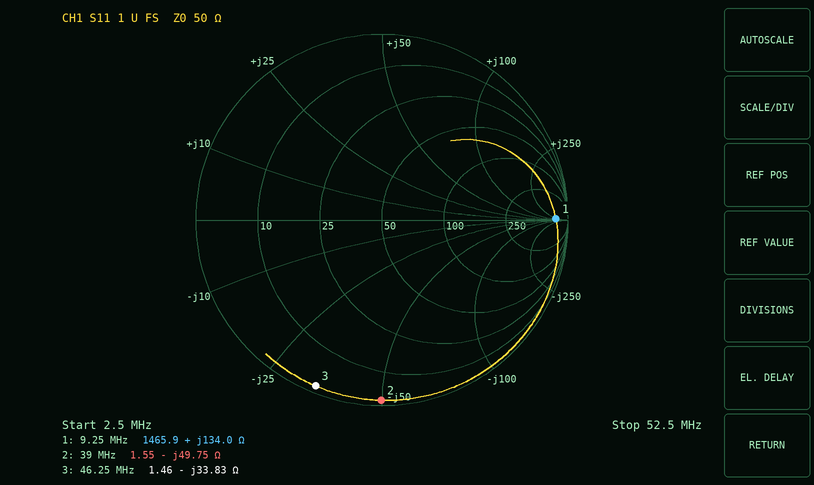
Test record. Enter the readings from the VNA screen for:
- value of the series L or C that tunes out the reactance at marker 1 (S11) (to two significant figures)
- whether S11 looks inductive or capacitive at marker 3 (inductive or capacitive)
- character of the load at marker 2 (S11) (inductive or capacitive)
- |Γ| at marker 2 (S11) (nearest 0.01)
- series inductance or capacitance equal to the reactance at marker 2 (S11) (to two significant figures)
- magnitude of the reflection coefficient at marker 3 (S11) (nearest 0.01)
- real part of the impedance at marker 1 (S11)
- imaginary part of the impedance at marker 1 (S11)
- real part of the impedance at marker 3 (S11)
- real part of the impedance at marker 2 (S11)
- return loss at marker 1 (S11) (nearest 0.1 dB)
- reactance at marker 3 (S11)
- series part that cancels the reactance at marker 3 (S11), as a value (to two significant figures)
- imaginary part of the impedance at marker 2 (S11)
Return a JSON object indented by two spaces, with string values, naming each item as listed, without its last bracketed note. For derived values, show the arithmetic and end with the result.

{
  "value of the series L or C that tunes out the reactance at marker 1 (S11)": "C = 1/(2π × 9.25 MHz × 134 Ω) ≈ 128 pF, so 130 pF to two significant figures",
  "whether S11 looks inductive or capacitive at marker 3": "capacitive",
  "character of the load at marker 2 (S11)": "capacitive",
  "|Γ| at marker 2 (S11)": "0.97",
  "series inductance or capacitance equal to the reactance at marker 2 (S11)": "C = 1/(2π × 39 MHz × 49.75 Ω) ≈ 82 pF",
  "magnitude of the reflection coefficient at marker 3 (S11)": "0.96",
  "real part of the impedance at marker 1": "1465.9 Ω",
  "imaginary part of the impedance at marker 1": "+134.0 Ω",
  "real part of the impedance at marker 3": "1.46 Ω",
  "real part of the impedance at marker 2": "1.55 Ω",
  "return loss at marker 1 (S11)": "0.6 dB",
  "reactance at marker 3": "-33.83 Ω",
  "series part that cancels the reactance at marker 3 (S11), as a value": "L = 33.83 Ω/(2π × 46.25 MHz) ≈ 116 nH, so 120 nH to two significant figures",
  "imaginary part of the impedance at marker 2": "-49.75 Ω"
}
